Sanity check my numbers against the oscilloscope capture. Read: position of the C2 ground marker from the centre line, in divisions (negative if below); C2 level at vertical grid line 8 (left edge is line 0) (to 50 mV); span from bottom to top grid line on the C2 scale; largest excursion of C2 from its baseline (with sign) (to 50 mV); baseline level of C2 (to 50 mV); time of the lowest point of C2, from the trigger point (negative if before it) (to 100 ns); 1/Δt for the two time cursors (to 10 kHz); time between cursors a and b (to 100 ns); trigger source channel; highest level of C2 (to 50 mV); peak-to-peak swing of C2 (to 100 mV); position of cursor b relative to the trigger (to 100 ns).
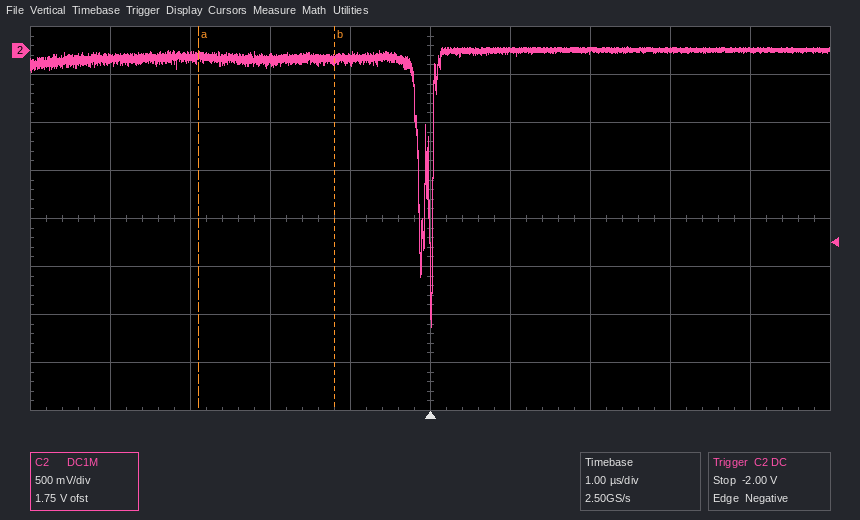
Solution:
+3.5 div
0 mV
4 V
-2.80 V
-50 mV
0.0 µs
590 kHz
1.7 µs
C2
50 mV
2.90 V
-1.2 µs
